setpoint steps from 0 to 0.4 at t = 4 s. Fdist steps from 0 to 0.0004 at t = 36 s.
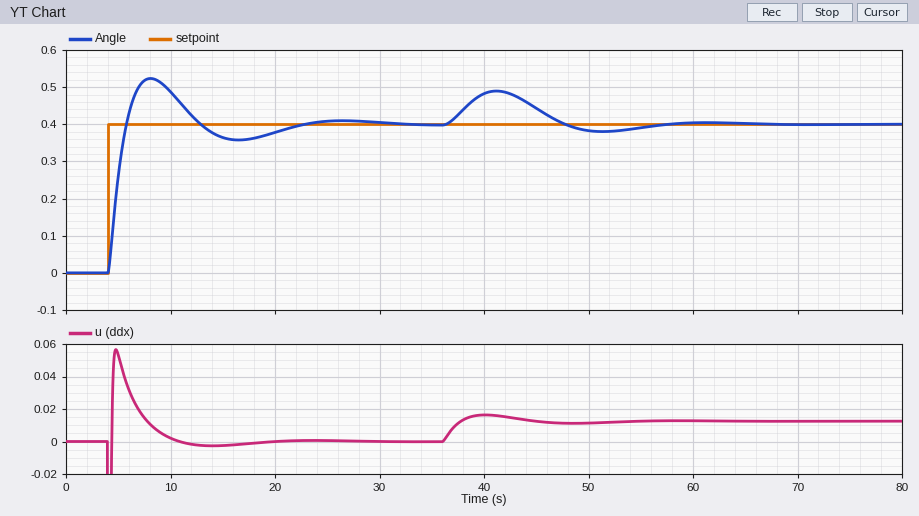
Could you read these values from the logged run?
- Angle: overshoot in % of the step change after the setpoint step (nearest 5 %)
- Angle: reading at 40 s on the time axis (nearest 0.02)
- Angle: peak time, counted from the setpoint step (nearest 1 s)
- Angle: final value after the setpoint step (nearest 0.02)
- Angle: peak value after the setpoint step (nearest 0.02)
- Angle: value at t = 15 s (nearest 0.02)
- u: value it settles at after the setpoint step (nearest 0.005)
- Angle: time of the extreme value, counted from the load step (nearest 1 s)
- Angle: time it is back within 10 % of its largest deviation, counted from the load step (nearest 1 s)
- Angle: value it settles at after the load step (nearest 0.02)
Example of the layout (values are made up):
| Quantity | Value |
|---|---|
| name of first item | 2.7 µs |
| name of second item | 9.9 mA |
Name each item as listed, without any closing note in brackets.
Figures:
| Quantity | Value |
|---|---|
| Angle: overshoot in % of the step change after the setpoint step | 30 % |
| Angle: reading at 40 s on the time axis | 0.48 |
| Angle: peak time, counted from the setpoint step | 4 s |
| Angle: final value after the setpoint step | 0.40 |
| Angle: peak value after the setpoint step | 0.52 |
| Angle: value at t = 15 s | 0.36 |
| u: value it settles at after the setpoint step | 0.000 |
| Angle: time of the extreme value, counted from the load step | 5 s |
| Angle: time it is back within 10 % of its largest deviation, counted from the load step | 19 s |
| Angle: value it settles at after the load step | 0.40 |
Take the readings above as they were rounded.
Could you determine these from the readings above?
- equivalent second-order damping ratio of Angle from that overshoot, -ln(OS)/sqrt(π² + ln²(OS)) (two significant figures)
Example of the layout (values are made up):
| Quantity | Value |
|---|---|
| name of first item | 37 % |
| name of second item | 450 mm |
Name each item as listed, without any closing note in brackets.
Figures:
| Quantity | Value |
|---|---|
| equivalent second-order damping ratio of Angle from that overshoot, -ln(OS)/sqrt(π² + ln²(OS)) | 0.36 |
